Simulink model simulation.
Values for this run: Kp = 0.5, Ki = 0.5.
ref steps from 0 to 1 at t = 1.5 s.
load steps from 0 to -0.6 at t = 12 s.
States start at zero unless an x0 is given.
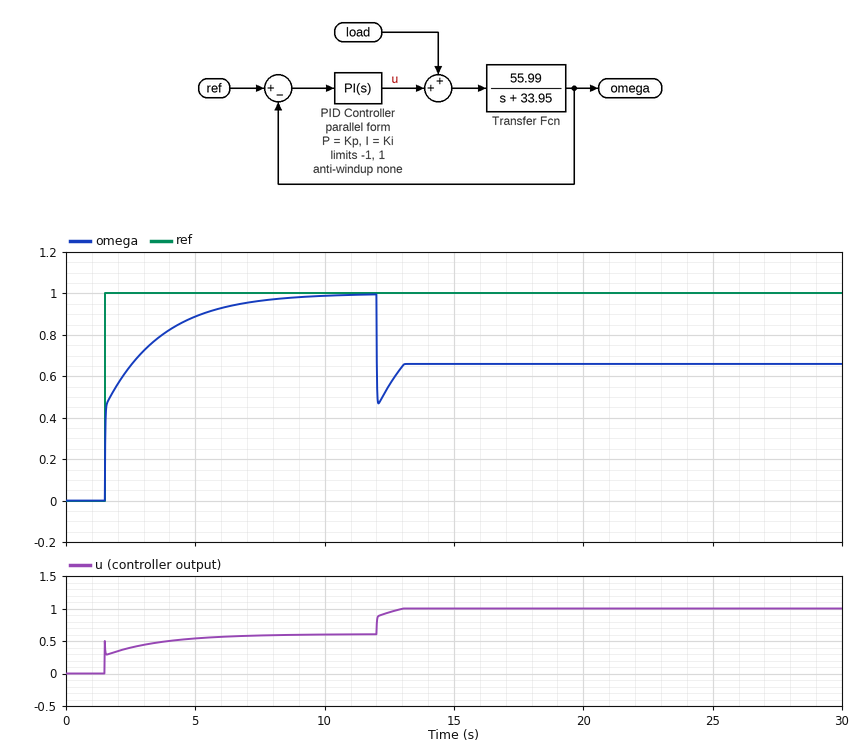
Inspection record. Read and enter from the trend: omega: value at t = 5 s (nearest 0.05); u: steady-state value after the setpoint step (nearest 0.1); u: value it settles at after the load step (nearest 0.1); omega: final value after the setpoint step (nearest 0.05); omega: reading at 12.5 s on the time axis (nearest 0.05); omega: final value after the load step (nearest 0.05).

0.90
0.6
1.0
1.00
0.55
0.65
